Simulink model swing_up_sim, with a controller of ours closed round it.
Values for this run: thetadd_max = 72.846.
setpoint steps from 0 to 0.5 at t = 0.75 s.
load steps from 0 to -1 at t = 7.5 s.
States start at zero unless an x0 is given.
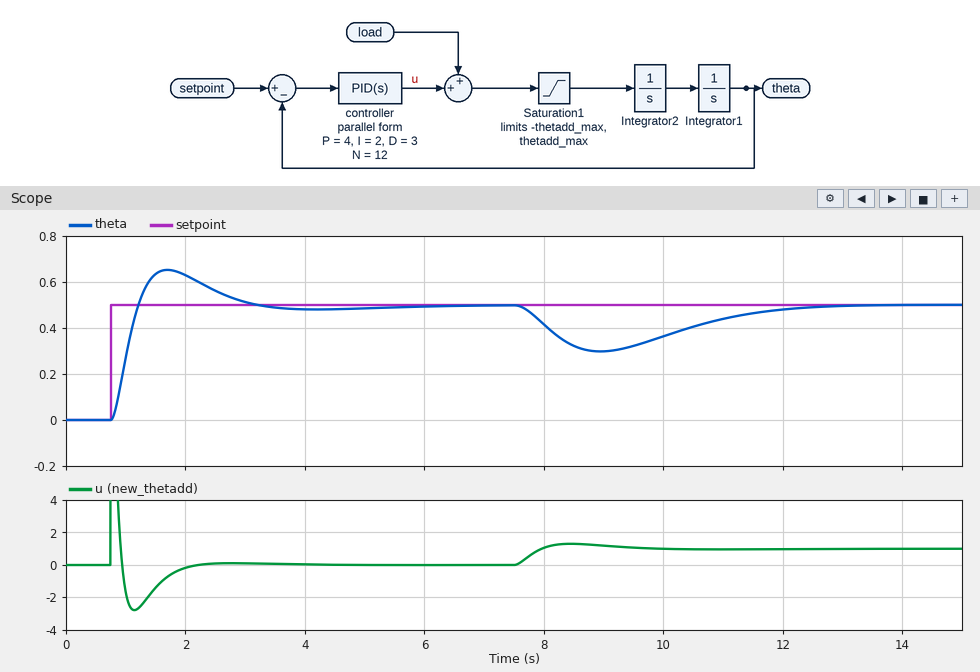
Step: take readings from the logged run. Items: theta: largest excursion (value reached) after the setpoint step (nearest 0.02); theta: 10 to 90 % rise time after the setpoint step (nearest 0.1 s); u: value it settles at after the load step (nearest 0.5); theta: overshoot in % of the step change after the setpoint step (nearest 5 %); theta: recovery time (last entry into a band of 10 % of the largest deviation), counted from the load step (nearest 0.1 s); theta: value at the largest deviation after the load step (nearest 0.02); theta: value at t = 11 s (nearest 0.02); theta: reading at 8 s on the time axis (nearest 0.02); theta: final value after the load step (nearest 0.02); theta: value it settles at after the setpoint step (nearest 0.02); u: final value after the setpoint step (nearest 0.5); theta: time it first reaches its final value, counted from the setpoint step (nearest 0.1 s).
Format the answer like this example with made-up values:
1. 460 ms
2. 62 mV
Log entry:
1. 0.66
2. 0.3 s
3. 1.0
4. 30 %
5. 4.5 s
6. 0.30
7. 0.44
8. 0.42
9. 0.50
10. 0.50
11. 0.0
12. 0.5 s
